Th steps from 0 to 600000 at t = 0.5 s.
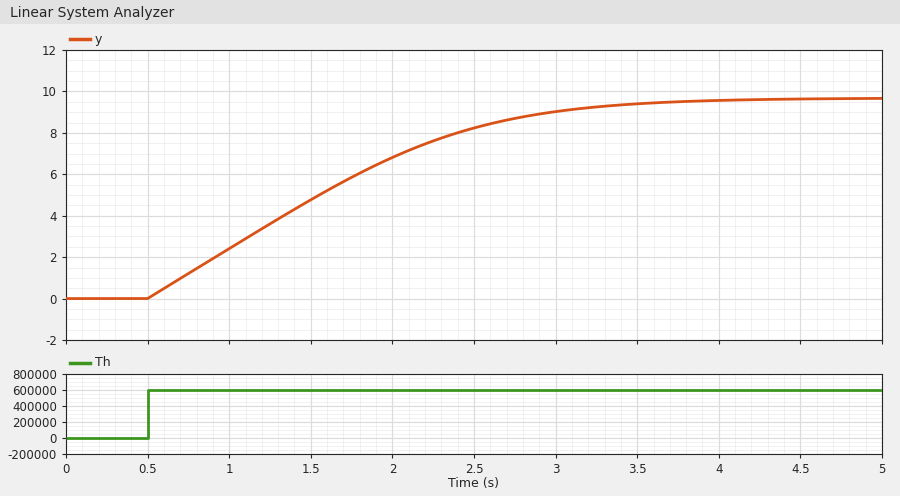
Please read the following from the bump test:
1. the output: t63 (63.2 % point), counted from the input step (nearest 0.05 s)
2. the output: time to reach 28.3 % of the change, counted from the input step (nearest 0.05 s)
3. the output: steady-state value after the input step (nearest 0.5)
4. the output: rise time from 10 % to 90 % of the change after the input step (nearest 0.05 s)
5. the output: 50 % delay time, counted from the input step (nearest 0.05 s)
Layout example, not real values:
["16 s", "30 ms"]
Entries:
["1.30 s", "0.55 s", "9.5", "2.05 s", "1.00 s"]
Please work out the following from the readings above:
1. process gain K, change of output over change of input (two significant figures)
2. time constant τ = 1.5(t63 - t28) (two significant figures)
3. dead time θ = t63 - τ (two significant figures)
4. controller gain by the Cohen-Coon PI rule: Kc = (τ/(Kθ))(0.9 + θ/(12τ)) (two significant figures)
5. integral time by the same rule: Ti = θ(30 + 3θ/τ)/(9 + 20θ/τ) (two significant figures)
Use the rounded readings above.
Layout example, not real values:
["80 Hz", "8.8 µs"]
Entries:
["0.000016", "1.1 s", "0.20 s", "310000", "0.48 s"]
